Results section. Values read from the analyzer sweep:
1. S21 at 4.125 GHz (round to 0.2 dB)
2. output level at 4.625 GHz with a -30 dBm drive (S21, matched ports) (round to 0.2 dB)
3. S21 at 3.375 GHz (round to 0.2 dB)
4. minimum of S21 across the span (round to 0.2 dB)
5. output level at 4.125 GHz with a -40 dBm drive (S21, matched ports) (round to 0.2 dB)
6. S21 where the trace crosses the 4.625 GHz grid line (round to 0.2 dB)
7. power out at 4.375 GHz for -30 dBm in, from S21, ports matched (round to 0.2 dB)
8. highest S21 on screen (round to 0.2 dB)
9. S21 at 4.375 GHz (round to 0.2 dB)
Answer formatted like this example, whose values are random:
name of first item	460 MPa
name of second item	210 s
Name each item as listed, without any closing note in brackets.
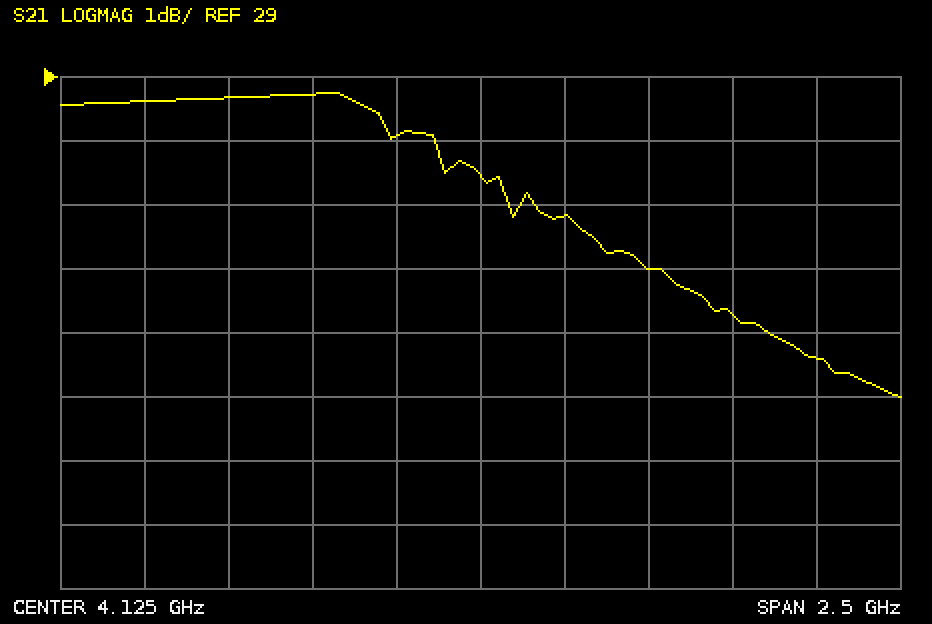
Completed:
S21 at 4.125 GHz	27.4 dB
output level at 4.625 GHz with a -30 dBm drive (S21, matched ports)	-4.0 dBm
S21 at 3.375 GHz	28.6 dB
minimum of S21 across the span	24.0 dB
output level at 4.125 GHz with a -40 dBm drive (S21, matched ports)	-12.6 dBm
S21 where the trace crosses the 4.625 GHz grid line	26.0 dB
power out at 4.375 GHz for -30 dBm in, from S21, ports matched	-3.2 dBm
highest S21 on screen	28.8 dB
S21 at 4.375 GHz	26.8 dB
